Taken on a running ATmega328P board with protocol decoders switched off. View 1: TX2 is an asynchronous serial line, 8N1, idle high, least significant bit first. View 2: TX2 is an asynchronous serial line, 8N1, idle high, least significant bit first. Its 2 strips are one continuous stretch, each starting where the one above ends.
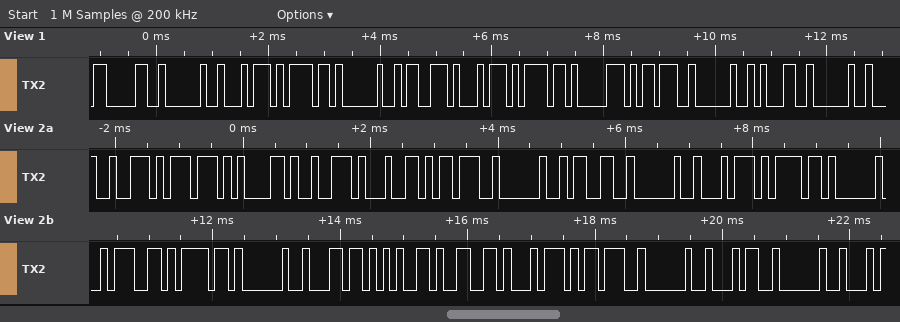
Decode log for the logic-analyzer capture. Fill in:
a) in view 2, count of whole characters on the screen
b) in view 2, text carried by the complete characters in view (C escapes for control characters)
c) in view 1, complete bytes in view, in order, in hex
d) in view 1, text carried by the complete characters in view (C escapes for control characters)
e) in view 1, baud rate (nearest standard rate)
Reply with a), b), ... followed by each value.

a) 23
b) "rward; 3 to go left; 4 "
c) 30 20 74 6F 20 73 74 6F 70 3B 20 31 20
d) "0 to stop; 1 "
e) 9600 baud
